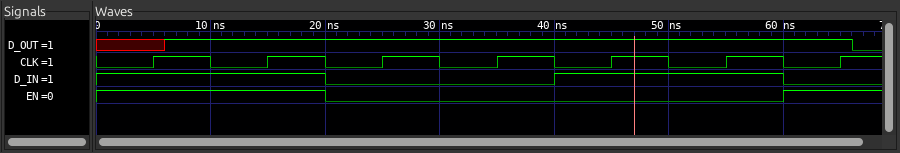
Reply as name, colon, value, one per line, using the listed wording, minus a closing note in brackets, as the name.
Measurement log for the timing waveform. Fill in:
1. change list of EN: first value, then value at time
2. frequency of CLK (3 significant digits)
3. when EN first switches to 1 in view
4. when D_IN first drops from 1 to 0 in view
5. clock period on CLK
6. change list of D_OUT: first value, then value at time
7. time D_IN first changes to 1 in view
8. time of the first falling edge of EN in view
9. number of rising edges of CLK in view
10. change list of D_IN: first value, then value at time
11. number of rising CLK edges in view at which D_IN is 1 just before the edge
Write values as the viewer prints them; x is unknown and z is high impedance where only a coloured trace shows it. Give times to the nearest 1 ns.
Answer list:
change list of EN: first value, then value at time: 1, 0 at 20 ns, 1 at 60 ns
frequency of CLK: 100 MHz
when EN first switches to 1 in view: 60 ns
when D_IN first drops from 1 to 0 in view: 20 ns
clock period on CLK: 10 ns
change list of D_OUT: first value, then value at time: x, 1 at 6 ns, 0 at 66 ns
time D_IN first changes to 1 in view: 40 ns
time of the first falling edge of EN in view: 20 ns
number of rising edges of CLK in view: 7
change list of D_IN: first value, then value at time: 1, 0 at 20 ns, 1 at 40 ns, 0 at 60 ns
number of rising CLK edges in view at which D_IN is 1 just before the edge: 4
